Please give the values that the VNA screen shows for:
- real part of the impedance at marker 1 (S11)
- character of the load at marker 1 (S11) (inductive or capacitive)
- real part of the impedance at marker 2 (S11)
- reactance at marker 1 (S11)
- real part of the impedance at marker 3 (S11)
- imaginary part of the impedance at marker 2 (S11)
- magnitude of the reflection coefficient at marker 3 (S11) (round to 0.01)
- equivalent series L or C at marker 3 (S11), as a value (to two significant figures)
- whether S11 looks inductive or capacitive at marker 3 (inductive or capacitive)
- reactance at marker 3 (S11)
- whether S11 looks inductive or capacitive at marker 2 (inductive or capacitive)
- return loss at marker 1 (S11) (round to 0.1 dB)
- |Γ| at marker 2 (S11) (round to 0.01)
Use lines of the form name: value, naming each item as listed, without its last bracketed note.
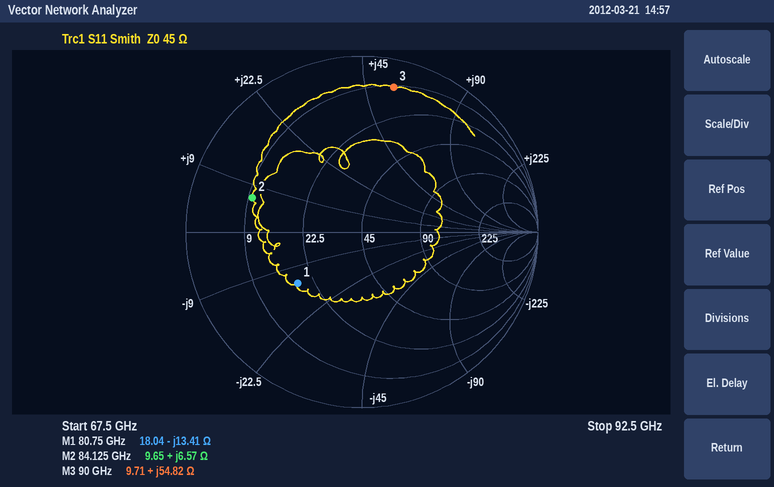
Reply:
real part of the impedance at marker 1: 18.04 Ω
character of the load at marker 1 (S11): capacitive
real part of the impedance at marker 2: 9.65 Ω
reactance at marker 1: -13.41 Ω
real part of the impedance at marker 3: 9.71 Ω
imaginary part of the impedance at marker 2: +6.57 Ω
magnitude of the reflection coefficient at marker 3 (S11): 0.84
equivalent series L or C at marker 3 (S11), as a value: 97 pH
whether S11 looks inductive or capacitive at marker 3: inductive
reactance at marker 3: +54.82 Ω
whether S11 looks inductive or capacitive at marker 2: inductive
return loss at marker 1 (S11): 6.6 dB
|Γ| at marker 2 (S11): 0.65
